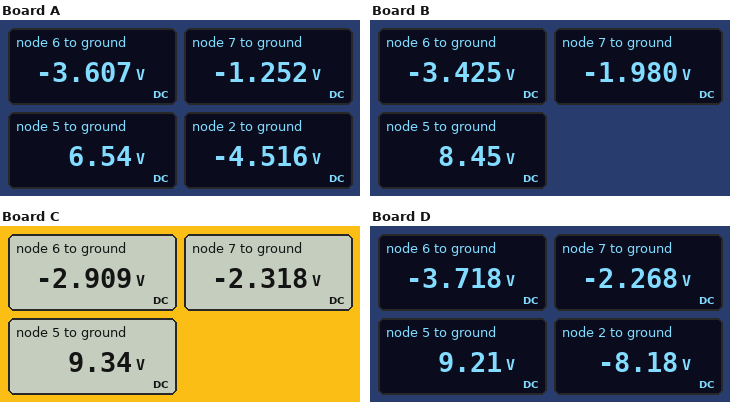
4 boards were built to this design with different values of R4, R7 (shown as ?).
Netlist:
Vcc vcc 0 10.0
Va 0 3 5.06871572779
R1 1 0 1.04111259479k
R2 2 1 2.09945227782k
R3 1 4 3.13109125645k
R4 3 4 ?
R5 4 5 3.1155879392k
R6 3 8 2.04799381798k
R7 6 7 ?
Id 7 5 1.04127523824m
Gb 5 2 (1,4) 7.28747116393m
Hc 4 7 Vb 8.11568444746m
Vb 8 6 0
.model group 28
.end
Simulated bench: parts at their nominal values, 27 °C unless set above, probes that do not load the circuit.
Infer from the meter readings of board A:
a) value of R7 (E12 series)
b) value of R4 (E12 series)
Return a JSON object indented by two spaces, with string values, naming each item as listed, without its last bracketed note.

{
  "value of R7": "3.3 kΩ",
  "value of R4": "5.6 kΩ"
}
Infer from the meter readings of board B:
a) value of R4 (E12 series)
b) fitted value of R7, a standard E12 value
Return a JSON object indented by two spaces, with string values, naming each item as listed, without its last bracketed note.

{
  "value of R4": "2.2 kΩ",
  "fitted value of R7, a standard E12 value": "1.8 kΩ"
}
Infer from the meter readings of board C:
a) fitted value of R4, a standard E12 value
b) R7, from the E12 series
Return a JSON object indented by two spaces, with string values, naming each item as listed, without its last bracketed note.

{
  "fitted value of R4, a standard E12 value": "1.8 kΩ",
  "R7, from the E12 series": "560 Ω"
}
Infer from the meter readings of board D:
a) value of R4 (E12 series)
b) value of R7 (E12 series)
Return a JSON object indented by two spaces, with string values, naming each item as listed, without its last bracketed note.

{
  "value of R4": "1.5 kΩ",
  "value of R7": "2.2 kΩ"
}
